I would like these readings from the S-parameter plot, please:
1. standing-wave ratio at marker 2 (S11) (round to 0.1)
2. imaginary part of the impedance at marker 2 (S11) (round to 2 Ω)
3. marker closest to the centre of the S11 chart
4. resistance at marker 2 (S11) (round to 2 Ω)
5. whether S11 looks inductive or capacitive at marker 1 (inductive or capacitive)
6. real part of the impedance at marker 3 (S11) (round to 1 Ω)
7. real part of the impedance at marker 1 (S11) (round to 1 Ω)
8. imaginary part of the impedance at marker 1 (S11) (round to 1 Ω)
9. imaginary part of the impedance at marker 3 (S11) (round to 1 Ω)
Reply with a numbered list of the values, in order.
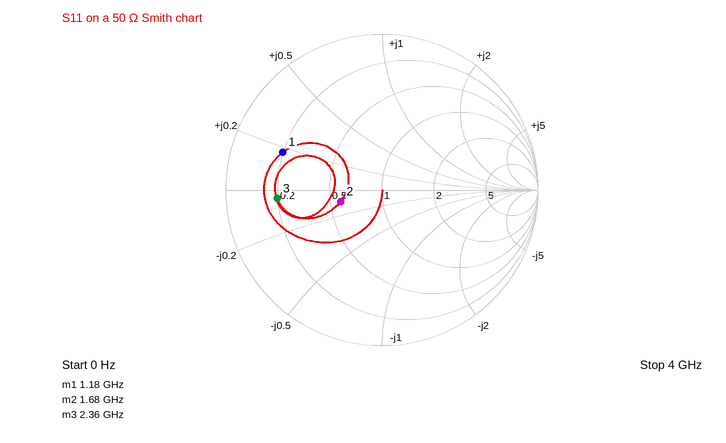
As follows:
1. 1.8
2. -4 Ω
3. marker 2
4. 28 Ω
5. inductive
6. 10 Ω
7. 10 Ω
8. +9 Ω
9. -2 Ω
